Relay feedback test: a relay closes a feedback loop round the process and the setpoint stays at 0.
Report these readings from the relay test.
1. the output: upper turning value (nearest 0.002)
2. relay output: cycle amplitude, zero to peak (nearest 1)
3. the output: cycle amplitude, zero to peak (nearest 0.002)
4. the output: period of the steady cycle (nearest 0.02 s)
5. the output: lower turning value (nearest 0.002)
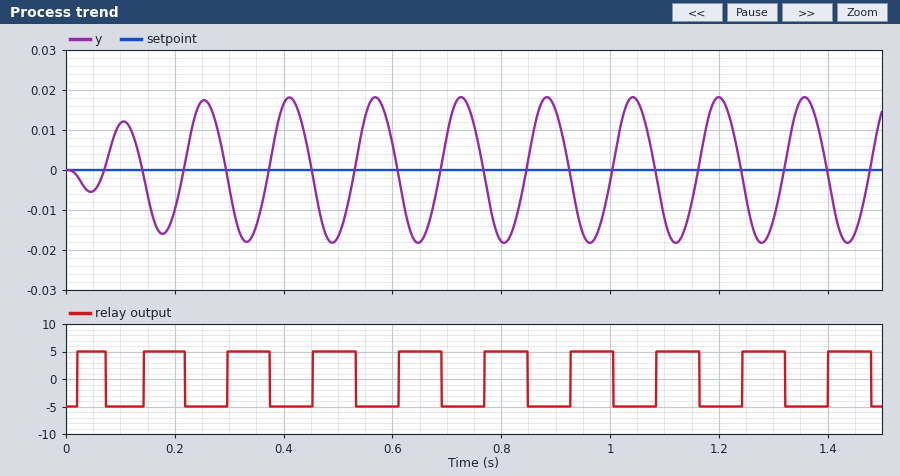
0.018
5
0.018
0.16 s
-0.018
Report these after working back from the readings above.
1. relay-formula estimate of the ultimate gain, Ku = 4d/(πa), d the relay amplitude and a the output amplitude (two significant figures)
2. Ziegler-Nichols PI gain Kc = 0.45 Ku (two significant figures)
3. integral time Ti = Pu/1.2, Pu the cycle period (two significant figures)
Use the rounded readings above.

350
160
0.13 s
